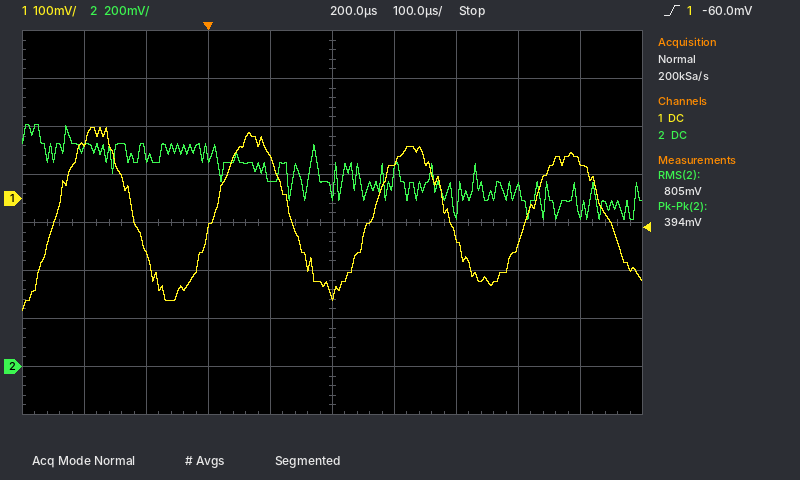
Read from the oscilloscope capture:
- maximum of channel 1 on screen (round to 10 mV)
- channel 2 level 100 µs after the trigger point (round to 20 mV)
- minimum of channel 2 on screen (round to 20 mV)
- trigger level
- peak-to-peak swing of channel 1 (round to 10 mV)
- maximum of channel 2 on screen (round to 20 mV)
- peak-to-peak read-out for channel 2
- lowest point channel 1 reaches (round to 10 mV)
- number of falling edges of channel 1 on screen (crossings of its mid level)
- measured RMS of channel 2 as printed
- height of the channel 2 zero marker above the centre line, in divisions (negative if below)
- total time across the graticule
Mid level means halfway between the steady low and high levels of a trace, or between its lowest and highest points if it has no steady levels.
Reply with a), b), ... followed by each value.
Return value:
a) 150 mV
b) 780 mV
c) 620 mV
d) -60.0 mV
e) 380 mV
f) 1.00 V
g) 394 mV
h) -230 mV
i) 4
j) 805 mV
k) -3.0 div
l) 1 ms
